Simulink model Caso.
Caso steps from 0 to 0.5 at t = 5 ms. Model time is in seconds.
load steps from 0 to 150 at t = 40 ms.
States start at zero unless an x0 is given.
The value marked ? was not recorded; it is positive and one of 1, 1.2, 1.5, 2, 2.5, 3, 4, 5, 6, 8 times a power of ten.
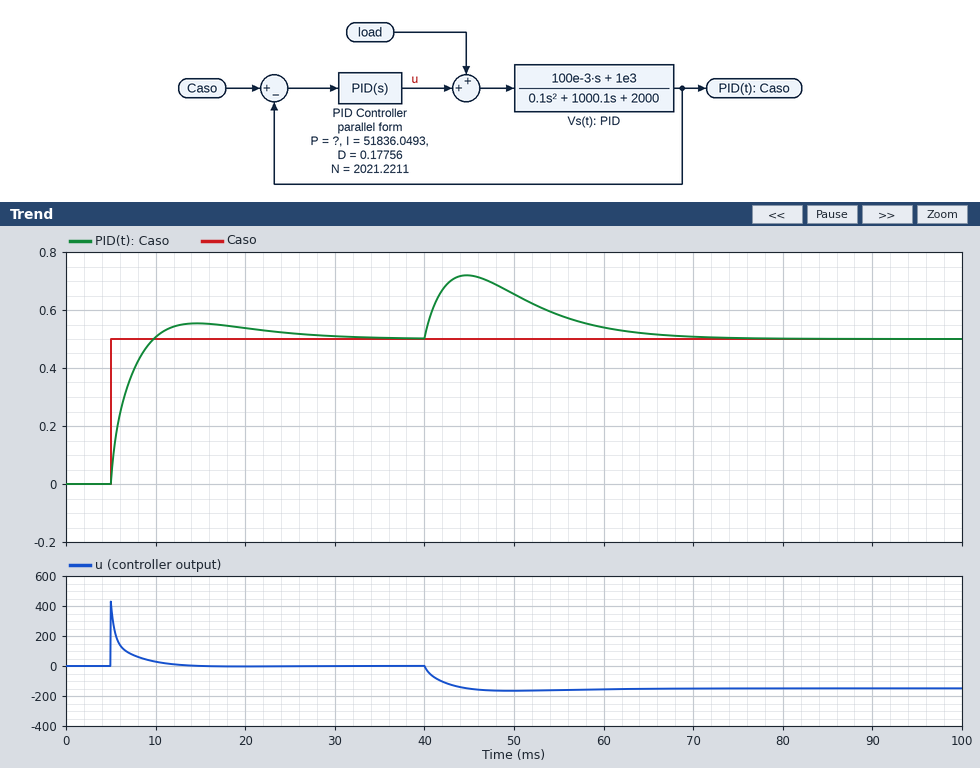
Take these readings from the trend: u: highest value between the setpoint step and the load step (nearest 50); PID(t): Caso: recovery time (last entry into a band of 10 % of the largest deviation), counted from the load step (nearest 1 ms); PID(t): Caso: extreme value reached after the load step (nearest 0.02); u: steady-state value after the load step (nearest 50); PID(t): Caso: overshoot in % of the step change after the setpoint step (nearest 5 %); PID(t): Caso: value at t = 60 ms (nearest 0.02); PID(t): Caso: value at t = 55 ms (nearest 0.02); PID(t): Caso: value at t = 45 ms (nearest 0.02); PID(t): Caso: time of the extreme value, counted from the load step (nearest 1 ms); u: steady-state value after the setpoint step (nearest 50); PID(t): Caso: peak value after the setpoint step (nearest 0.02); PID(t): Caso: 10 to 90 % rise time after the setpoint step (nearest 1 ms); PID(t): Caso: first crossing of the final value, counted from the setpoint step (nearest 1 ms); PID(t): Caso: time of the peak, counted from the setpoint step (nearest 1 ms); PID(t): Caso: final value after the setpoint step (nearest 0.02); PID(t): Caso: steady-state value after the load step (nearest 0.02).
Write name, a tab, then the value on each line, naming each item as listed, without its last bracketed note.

u: highest value between the setpoint step and the load step	450
PID(t): Caso: recovery time (last entry into a band of 10 % of the largest deviation), counted from the load step	24 ms
PID(t): Caso: extreme value reached after the load step	0.72
u: steady-state value after the load step	-150
PID(t): Caso: overshoot in % of the step change after the setpoint step	10 %
PID(t): Caso: value at t = 60 ms	0.54
PID(t): Caso: value at t = 55 ms	0.58
PID(t): Caso: value at t = 45 ms	0.72
PID(t): Caso: time of the extreme value, counted from the load step	5 ms
u: steady-state value after the setpoint step	0
PID(t): Caso: peak value after the setpoint step	0.56
PID(t): Caso: 10 to 90 % rise time after the setpoint step	3 ms
PID(t): Caso: first crossing of the final value, counted from the setpoint step	5 ms
PID(t): Caso: time of the peak, counted from the setpoint step	10 ms
PID(t): Caso: final value after the setpoint step	0.50
PID(t): Caso: steady-state value after the load step	0.50
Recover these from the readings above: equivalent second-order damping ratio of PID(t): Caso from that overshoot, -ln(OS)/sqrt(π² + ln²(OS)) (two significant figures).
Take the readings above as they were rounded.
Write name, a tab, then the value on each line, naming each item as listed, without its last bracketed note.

equivalent second-order damping ratio of PID(t): Caso from that overshoot, -ln(OS)/sqrt(π² + ln²(OS))	0.59
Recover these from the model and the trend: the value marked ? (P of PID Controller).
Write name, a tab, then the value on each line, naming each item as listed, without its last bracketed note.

the value marked ?	500
